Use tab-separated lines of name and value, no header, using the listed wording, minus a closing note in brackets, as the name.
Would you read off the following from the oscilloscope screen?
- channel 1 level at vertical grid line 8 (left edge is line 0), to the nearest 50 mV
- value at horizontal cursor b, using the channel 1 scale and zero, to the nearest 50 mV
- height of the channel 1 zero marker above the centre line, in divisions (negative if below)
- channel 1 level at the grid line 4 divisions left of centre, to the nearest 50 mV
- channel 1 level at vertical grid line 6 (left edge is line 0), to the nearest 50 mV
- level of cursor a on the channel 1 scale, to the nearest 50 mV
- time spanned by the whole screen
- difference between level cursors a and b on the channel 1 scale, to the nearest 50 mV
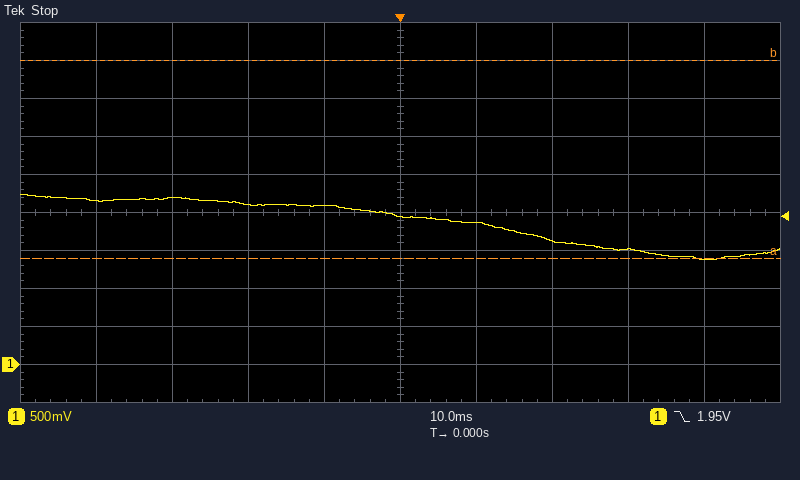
channel 1 level at vertical grid line 8 (left edge is line 0), to the nearest 50 mV	1.50 V
value at horizontal cursor b, using the channel 1 scale and zero, to the nearest 50 mV	4.00 V
height of the channel 1 zero marker above the centre line, in divisions	-4.0 div
channel 1 level at the grid line 4 divisions left of centre, to the nearest 50 mV	2.15 V
channel 1 level at vertical grid line 6 (left edge is line 0), to the nearest 50 mV	1.85 V
level of cursor a on the channel 1 scale, to the nearest 50 mV	1.40 V
time spanned by the whole screen	100 ms
difference between level cursors a and b on the channel 1 scale, to the nearest 50 mV	2.60 V
